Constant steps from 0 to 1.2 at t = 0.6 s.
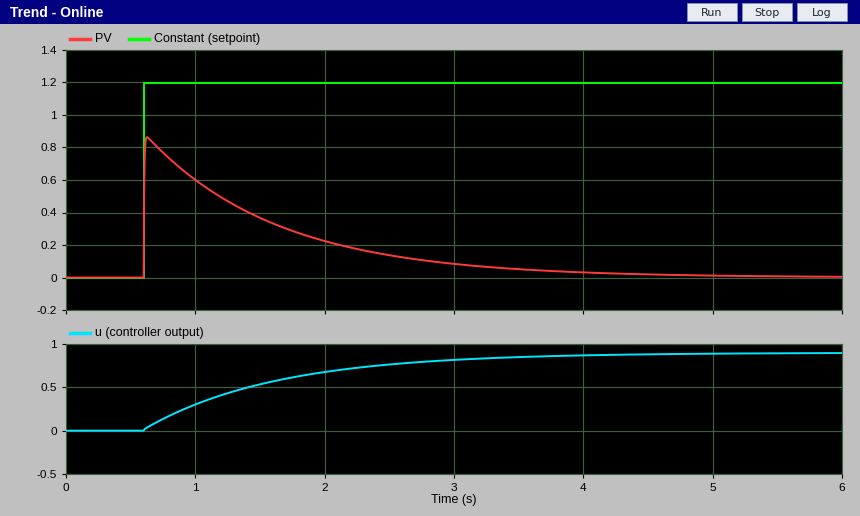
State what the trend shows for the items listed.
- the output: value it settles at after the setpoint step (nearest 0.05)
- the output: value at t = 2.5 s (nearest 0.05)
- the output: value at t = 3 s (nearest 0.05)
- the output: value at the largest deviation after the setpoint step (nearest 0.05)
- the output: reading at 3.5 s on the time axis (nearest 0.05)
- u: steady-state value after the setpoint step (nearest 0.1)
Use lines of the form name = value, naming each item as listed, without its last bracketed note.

the output: value it settles at after the setpoint step = 0.00
the output: value at t = 2.5 s = 0.15
the output: value at t = 3 s = 0.10
the output: value at the largest deviation after the setpoint step = 0.85
the output: reading at 3.5 s on the time axis = 0.05
u: steady-state value after the setpoint step = 0.9
